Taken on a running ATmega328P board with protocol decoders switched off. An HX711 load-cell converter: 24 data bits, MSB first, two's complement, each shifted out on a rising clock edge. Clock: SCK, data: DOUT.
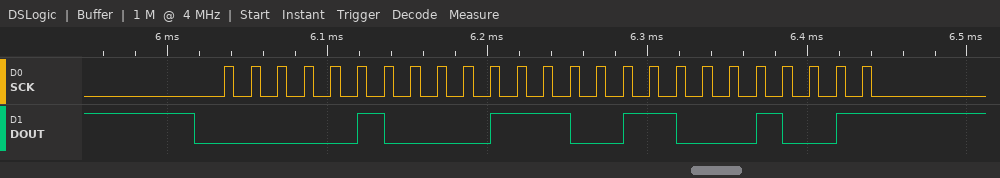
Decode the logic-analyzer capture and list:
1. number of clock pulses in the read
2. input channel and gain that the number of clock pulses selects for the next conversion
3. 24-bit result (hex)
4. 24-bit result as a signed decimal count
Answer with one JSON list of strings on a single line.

["25", "channel A, gain 128", "0x043989", "276873"]
